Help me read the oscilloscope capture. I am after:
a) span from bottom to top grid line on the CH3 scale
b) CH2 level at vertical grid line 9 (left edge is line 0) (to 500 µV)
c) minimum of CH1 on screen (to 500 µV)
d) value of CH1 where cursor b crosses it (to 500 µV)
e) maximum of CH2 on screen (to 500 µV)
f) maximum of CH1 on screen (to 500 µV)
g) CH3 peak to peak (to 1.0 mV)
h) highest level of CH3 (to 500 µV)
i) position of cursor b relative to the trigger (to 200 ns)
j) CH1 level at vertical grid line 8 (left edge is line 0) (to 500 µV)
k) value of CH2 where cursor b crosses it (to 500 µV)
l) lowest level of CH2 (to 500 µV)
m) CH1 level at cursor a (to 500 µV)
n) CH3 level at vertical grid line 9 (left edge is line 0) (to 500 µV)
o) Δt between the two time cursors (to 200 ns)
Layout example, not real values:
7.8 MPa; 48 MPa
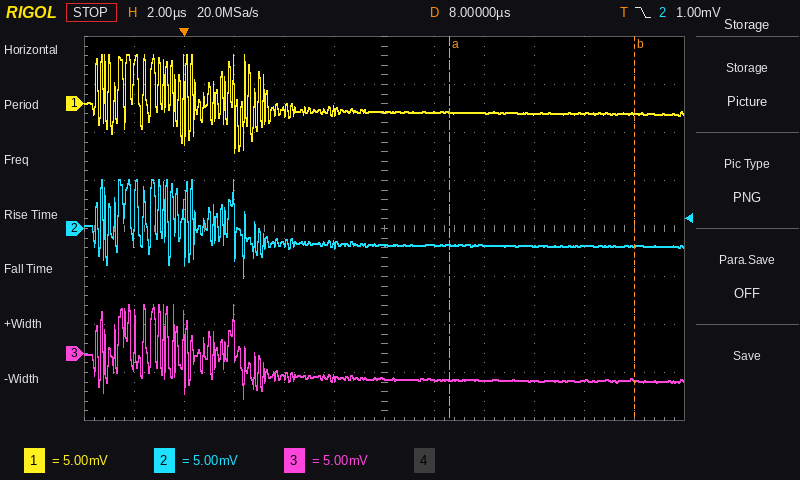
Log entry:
40 mV; -2.0 mV; -5.0 mV; -1.0 mV; 5.0 mV; 5.0 mV; 10.0 mV; 5.0 mV; +18.0 µs; -1.0 mV; -2.0 mV; -5.0 mV; -1.0 mV; -3.0 mV; 7.4 µs
